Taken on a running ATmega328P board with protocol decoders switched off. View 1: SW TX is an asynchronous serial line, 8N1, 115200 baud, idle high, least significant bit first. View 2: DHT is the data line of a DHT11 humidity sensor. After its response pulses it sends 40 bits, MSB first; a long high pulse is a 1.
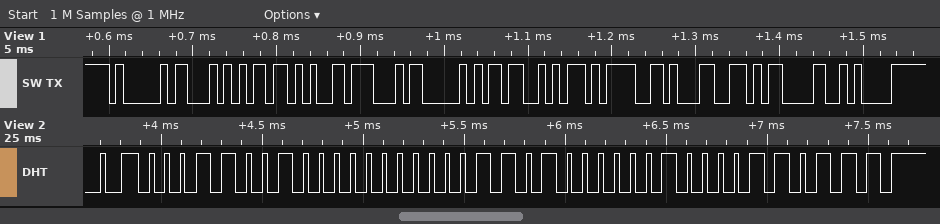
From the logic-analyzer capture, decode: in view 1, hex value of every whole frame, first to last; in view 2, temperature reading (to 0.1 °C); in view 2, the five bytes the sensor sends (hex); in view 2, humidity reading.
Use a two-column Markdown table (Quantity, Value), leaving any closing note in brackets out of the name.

| Quantity | Value |
|---|---|
| in view 1, hex value of every whole frame, first to last | 0x41 0x54 0x2B 0x47 0x50 0x53 0x3D 0x31 0x0D 0x0A |
| in view 2, temperature reading | 26.4 °C |
| in view 2, the five bytes the sensor sends | 19 00 1A 04 37 |
| in view 2, humidity reading | 25 % |
